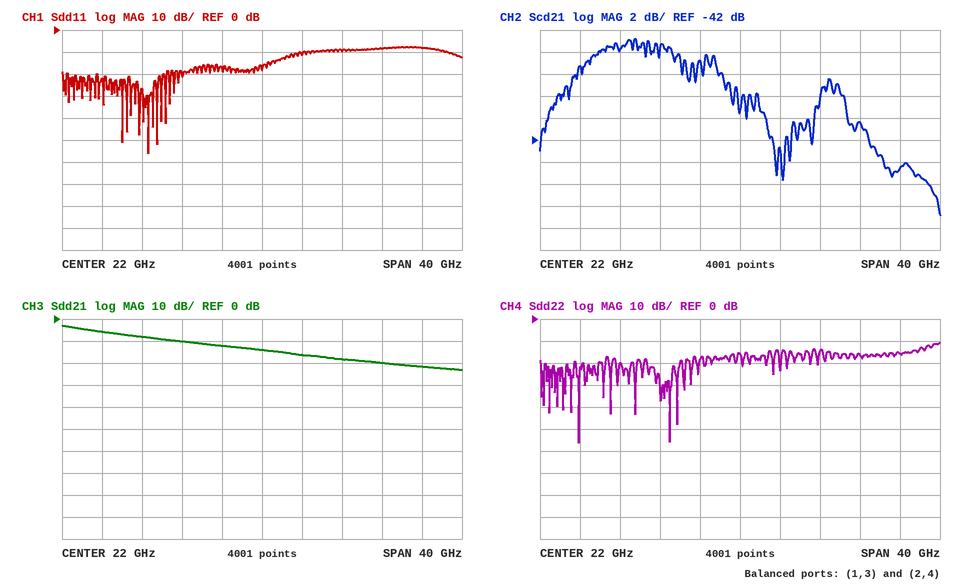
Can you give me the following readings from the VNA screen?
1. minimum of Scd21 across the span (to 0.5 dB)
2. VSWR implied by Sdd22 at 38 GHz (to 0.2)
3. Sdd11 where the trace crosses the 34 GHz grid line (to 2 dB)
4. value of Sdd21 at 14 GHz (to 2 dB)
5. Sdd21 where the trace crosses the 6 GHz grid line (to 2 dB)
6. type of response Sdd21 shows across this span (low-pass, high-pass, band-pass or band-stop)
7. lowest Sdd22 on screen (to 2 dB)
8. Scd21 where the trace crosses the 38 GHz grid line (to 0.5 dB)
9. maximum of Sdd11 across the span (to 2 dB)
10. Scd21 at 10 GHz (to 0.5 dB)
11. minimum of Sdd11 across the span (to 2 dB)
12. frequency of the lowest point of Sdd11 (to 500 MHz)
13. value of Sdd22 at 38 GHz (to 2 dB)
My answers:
-49.0 dB
1.4
-8 dB
-10 dB
-6 dB
low-pass
-56 dB
-44.5 dB
-8 dB
-34.0 dB
-56 dB
10.5 GHz
-16 dB
